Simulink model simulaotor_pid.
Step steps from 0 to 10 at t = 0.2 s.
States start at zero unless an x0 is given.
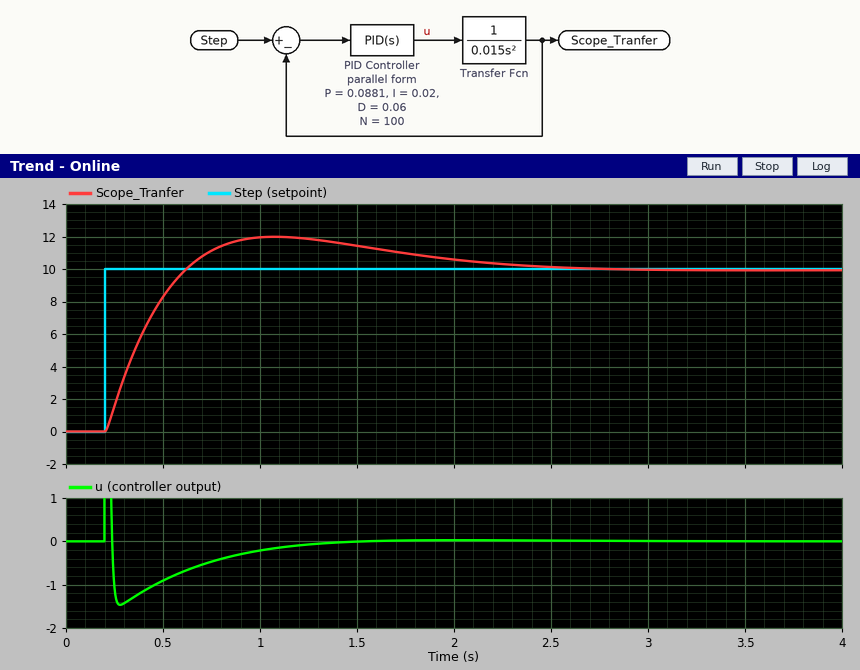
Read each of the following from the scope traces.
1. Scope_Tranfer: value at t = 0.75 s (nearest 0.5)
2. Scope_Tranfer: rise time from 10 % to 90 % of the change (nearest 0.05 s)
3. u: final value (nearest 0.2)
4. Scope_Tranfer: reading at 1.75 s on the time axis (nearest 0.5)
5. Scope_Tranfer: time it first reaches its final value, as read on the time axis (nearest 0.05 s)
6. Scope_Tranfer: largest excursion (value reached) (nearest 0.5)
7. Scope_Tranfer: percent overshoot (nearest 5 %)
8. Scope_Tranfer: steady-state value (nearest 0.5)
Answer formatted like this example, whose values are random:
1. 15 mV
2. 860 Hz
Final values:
1. 11.0
2. 0.30 s
3. 0.0
4. 11.0
5. 0.60 s
6. 12.0
7. 20 %
8. 10.0
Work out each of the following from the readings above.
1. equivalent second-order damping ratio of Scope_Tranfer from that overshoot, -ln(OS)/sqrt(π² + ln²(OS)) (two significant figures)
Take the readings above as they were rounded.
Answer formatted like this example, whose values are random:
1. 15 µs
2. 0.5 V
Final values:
1. 0.46
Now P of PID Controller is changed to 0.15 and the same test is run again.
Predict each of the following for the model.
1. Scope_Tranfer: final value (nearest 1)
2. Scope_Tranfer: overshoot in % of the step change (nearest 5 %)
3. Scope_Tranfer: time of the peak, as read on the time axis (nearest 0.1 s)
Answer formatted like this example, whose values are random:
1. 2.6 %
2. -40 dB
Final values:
1. 10
2. 25 %
3. 0.9 s
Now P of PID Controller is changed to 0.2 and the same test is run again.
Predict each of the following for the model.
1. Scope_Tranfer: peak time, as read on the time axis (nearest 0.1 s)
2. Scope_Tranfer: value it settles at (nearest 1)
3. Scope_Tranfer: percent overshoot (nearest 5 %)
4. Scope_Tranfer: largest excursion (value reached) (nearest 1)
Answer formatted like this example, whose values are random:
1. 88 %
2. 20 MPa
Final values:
1. 0.8 s
2. 10
3. 30 %
4. 13
